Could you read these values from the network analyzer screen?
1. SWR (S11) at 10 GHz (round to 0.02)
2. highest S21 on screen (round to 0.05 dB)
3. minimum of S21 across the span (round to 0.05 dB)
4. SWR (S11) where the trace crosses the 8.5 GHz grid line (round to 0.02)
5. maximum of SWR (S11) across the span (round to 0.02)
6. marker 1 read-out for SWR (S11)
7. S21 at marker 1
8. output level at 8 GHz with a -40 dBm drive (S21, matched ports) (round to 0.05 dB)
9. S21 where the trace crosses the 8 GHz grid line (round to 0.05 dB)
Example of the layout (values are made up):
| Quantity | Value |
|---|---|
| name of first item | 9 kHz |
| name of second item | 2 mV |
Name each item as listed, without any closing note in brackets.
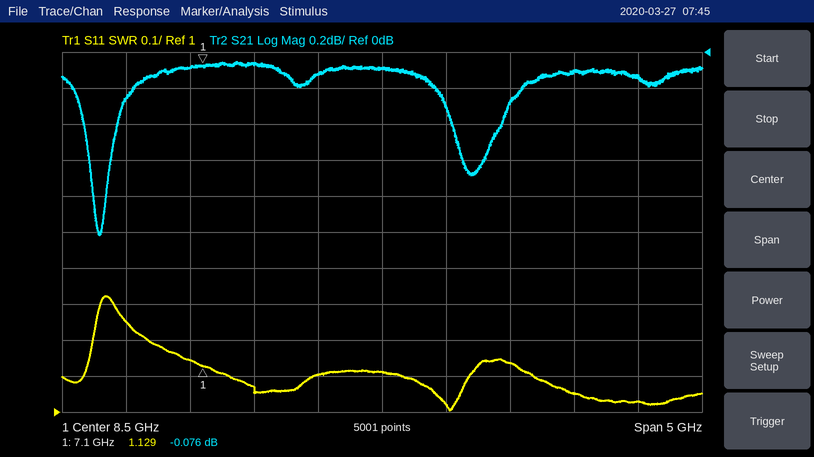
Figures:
| Quantity | Value |
|---|---|
| SWR (S11) at 10 GHz | 1.06 |
| highest S21 on screen | -0.05 dB |
| minimum of S21 across the span | -1.00 dB |
| SWR (S11) where the trace crosses the 8.5 GHz grid line | 1.12 |
| maximum of SWR (S11) across the span | 1.32 |
| marker 1 read-out for SWR | 1.129 |
| S21 at marker 1 | -0.076 dB |
| output level at 8 GHz with a -40 dBm drive (S21, matched ports) | -40.10 dBm |
| S21 where the trace crosses the 8 GHz grid line | -0.10 dB |
